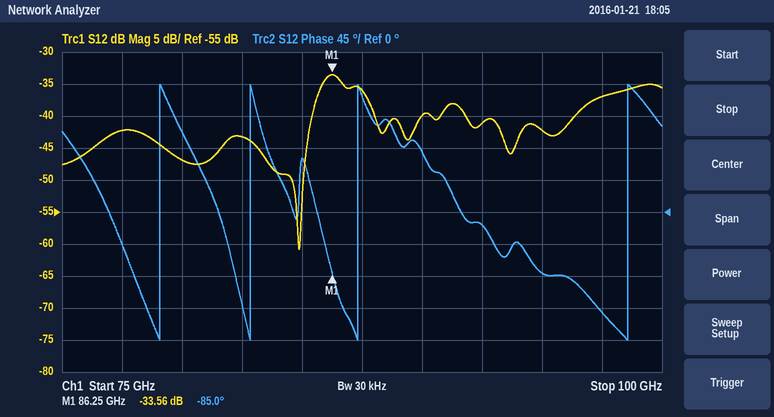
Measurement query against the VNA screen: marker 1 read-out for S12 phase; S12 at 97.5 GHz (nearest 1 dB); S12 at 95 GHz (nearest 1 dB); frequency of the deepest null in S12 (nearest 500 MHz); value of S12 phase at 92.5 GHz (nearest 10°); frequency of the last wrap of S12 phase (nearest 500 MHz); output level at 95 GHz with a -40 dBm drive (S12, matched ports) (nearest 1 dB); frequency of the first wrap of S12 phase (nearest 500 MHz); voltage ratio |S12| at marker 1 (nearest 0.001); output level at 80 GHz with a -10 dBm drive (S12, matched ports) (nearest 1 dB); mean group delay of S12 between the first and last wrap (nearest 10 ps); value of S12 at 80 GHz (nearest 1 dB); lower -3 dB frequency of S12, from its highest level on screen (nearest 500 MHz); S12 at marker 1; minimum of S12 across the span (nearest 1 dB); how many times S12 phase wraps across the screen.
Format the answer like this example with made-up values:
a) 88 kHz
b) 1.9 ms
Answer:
a) -85.0°
b) -37 dB
c) -42 dB
d) 85.0 GHz
e) -20°
f) 98.5 GHz
g) -82 dBm
h) 79.0 GHz
i) 0.021
j) -57 dBm
k) 150 ps
l) -47 dB
m) 85.5 GHz
n) -33.56 dB
o) -61 dB
p) 4
